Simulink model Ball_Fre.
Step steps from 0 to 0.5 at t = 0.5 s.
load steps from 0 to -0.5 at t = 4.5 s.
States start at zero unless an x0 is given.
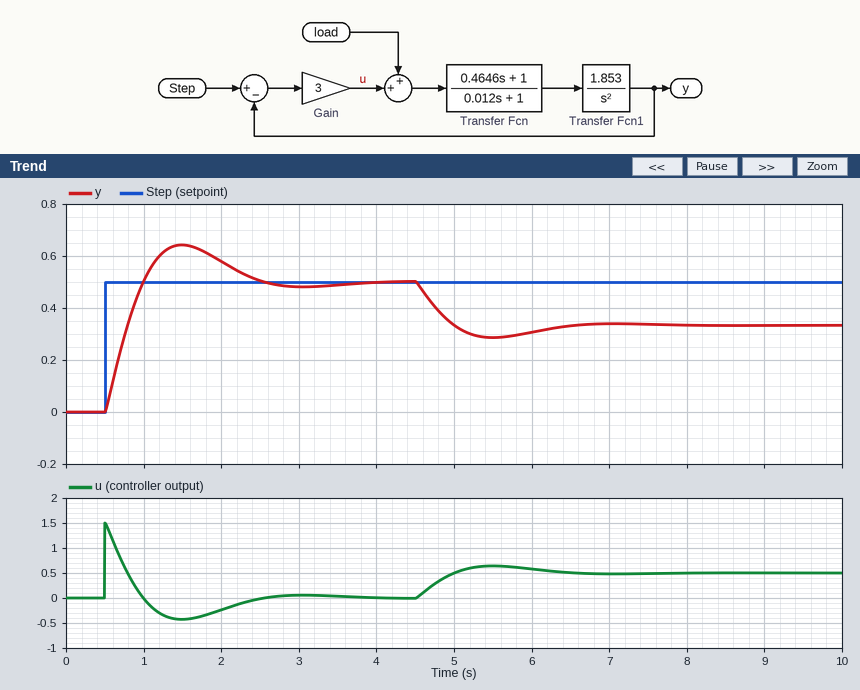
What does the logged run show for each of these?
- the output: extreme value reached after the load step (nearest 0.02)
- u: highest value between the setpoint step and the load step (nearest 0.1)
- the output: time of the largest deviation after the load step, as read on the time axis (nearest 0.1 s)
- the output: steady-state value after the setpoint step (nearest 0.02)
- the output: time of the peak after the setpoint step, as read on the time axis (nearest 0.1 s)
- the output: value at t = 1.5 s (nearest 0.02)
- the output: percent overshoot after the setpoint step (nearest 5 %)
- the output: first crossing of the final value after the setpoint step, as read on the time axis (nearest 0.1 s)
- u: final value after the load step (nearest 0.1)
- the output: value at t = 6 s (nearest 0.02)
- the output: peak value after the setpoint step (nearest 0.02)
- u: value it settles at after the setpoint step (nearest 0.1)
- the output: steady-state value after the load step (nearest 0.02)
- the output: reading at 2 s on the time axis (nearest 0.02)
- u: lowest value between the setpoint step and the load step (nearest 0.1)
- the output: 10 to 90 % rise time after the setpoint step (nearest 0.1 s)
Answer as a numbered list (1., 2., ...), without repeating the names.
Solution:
1. 0.28
2. 1.5
3. 5.5 s
4. 0.50
5. 1.5 s
6. 0.64
7. 30 %
8. 1.0 s
9. 0.5
10. 0.30
11. 0.64
12. 0.0
13. 0.34
14. 0.58
15. -0.4
16. 0.4 s
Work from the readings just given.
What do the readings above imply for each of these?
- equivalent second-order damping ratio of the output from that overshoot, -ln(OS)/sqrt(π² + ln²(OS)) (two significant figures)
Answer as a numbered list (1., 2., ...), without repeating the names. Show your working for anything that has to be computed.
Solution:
1. ln(0.3) = -1.204; 1.204 / sqrt(9.870 + 1.450) = 0.36
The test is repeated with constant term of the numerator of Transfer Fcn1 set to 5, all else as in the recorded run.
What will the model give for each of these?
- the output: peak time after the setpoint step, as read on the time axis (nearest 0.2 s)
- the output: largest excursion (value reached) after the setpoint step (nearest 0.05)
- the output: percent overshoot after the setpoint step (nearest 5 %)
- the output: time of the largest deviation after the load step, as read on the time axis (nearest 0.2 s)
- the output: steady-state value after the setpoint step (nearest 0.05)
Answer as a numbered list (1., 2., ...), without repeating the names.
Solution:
1. 1.0 s
2. 0.60
3. 15 %
4. 5.0 s
5. 0.50
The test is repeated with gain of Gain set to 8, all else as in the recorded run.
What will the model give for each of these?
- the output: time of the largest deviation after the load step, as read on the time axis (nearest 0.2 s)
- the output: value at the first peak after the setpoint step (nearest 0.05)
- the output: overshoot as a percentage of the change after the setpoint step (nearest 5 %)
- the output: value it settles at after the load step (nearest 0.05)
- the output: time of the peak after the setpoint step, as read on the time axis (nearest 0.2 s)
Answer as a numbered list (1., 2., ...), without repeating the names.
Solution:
1. 5.0 s
2. 0.60
3. 15 %
4. 0.45
5. 1.0 s
